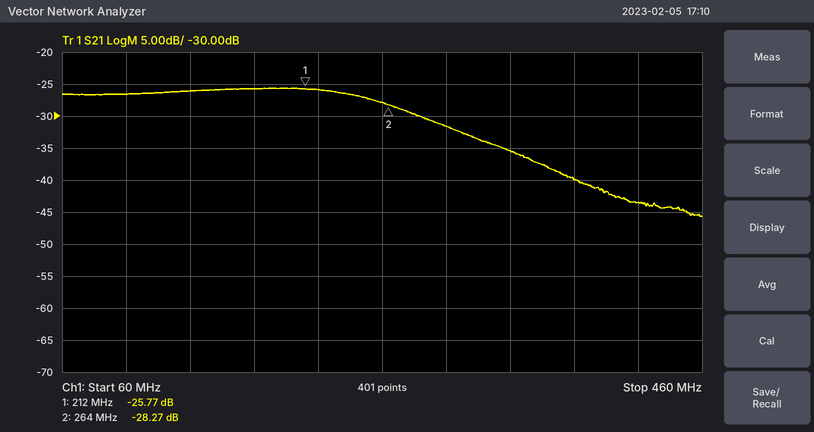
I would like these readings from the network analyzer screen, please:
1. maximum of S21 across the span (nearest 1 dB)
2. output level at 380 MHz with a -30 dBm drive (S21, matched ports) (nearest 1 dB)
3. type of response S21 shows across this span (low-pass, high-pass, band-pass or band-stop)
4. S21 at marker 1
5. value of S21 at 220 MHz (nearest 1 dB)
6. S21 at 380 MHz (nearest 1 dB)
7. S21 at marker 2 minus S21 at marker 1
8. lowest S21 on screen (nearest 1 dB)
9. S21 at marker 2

-26 dB
-70 dBm
low-pass
-25.77 dB
-26 dB
-40 dB
-2.50 dB
-46 dB
-28.27 dB
